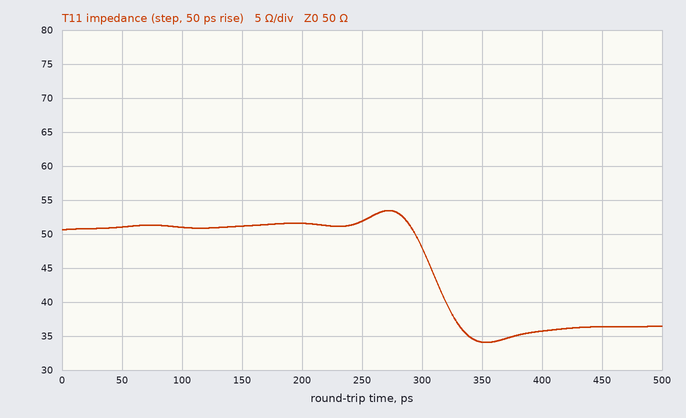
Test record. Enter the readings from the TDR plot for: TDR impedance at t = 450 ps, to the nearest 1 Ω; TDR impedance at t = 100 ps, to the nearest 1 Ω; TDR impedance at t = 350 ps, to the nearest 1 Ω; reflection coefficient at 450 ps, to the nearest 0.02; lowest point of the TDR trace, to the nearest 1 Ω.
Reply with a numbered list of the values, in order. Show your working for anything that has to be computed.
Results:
1. 36 Ω
2. 51 Ω
3. 34 Ω
4. (36 − 50)/(36 + 50) ≈ -0.16
5. 34 Ω
